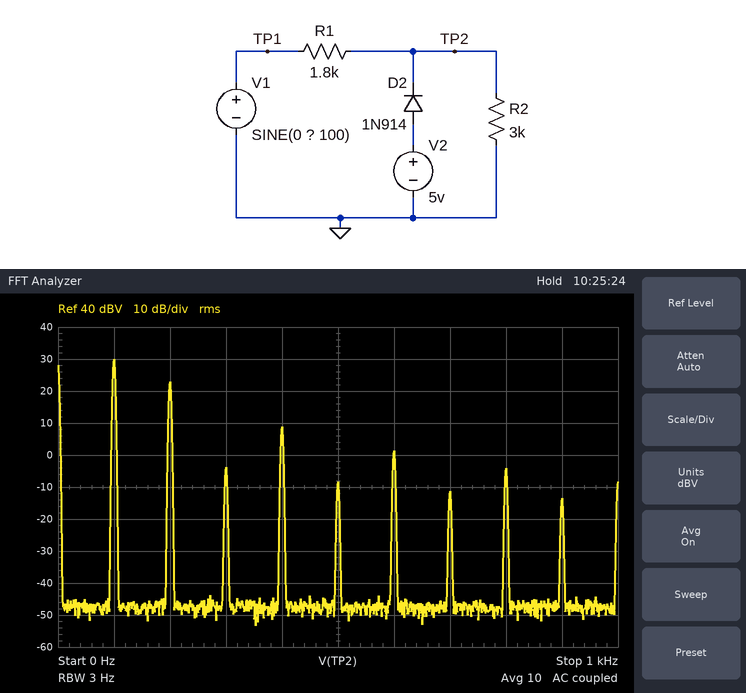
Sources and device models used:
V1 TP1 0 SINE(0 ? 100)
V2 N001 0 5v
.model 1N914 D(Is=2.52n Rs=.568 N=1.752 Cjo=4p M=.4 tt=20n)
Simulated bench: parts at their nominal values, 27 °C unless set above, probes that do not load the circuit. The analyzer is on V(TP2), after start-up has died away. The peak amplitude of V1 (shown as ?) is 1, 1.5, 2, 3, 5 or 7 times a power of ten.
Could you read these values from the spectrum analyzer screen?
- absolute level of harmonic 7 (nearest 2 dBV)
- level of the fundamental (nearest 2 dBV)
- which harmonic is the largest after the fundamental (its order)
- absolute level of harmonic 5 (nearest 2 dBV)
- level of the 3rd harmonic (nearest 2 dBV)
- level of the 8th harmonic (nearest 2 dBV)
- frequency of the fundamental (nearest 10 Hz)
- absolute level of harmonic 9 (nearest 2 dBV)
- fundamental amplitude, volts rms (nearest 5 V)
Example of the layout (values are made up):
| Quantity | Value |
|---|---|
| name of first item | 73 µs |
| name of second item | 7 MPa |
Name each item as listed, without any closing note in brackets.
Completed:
| Quantity | Value |
|---|---|
| absolute level of harmonic 7 | -12 dBV |
| level of the fundamental | 30 dBV |
| which harmonic is the largest after the fundamental | 2 |
| absolute level of harmonic 5 | -8 dBV |
| level of the 3rd harmonic | -4 dBV |
| level of the 8th harmonic | -4 dBV |
| frequency of the fundamental | 100 Hz |
| absolute level of harmonic 9 | -14 dBV |
| fundamental amplitude, volts rms | 30 V |
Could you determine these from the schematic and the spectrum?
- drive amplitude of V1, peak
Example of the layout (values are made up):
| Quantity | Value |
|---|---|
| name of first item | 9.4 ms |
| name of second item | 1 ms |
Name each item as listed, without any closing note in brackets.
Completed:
| Quantity | Value |
|---|---|
| drive amplitude of V1, peak | 150 V |
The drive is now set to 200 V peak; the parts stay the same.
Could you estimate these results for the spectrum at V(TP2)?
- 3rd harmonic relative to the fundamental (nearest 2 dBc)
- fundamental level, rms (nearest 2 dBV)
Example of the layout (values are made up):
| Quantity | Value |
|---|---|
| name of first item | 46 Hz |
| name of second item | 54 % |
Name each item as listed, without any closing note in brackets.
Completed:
| Quantity | Value |
|---|---|
| 3rd harmonic relative to the fundamental | -36 dBc |
| fundamental level, rms | 32 dBV |
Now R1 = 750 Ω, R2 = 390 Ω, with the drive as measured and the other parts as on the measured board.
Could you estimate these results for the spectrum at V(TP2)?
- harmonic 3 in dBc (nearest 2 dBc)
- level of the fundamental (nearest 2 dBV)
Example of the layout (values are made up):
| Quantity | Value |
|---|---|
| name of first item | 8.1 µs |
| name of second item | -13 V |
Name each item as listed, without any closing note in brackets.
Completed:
| Quantity | Value |
|---|---|
| harmonic 3 in dBc | -28 dBc |
| level of the fundamental | 24 dBV |
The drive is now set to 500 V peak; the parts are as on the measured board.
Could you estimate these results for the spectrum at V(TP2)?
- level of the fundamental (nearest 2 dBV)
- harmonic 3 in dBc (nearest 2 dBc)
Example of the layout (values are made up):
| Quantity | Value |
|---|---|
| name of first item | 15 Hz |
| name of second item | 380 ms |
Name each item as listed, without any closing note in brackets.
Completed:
| Quantity | Value |
|---|---|
| level of the fundamental | 40 dBV |
| harmonic 3 in dBc | -44 dBc |
